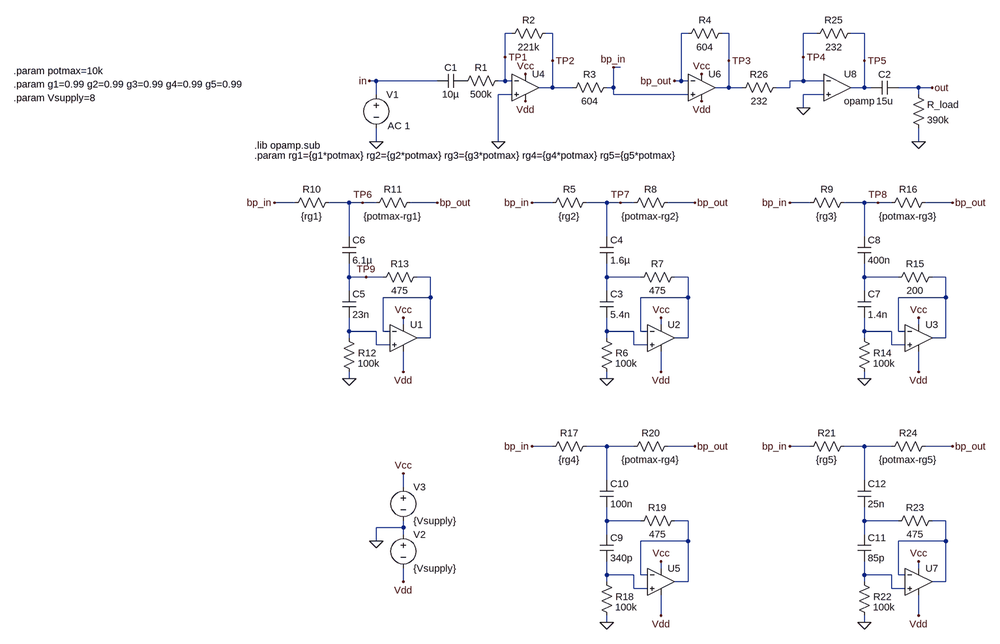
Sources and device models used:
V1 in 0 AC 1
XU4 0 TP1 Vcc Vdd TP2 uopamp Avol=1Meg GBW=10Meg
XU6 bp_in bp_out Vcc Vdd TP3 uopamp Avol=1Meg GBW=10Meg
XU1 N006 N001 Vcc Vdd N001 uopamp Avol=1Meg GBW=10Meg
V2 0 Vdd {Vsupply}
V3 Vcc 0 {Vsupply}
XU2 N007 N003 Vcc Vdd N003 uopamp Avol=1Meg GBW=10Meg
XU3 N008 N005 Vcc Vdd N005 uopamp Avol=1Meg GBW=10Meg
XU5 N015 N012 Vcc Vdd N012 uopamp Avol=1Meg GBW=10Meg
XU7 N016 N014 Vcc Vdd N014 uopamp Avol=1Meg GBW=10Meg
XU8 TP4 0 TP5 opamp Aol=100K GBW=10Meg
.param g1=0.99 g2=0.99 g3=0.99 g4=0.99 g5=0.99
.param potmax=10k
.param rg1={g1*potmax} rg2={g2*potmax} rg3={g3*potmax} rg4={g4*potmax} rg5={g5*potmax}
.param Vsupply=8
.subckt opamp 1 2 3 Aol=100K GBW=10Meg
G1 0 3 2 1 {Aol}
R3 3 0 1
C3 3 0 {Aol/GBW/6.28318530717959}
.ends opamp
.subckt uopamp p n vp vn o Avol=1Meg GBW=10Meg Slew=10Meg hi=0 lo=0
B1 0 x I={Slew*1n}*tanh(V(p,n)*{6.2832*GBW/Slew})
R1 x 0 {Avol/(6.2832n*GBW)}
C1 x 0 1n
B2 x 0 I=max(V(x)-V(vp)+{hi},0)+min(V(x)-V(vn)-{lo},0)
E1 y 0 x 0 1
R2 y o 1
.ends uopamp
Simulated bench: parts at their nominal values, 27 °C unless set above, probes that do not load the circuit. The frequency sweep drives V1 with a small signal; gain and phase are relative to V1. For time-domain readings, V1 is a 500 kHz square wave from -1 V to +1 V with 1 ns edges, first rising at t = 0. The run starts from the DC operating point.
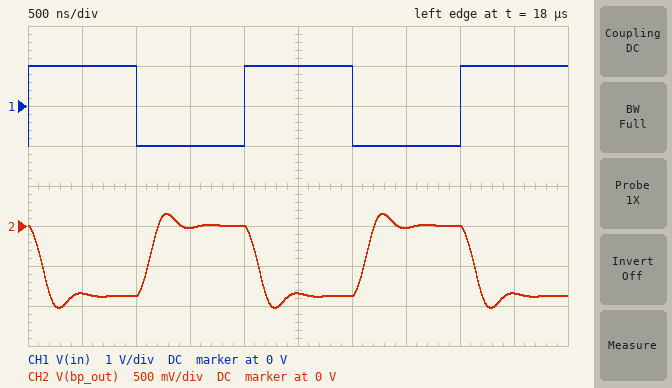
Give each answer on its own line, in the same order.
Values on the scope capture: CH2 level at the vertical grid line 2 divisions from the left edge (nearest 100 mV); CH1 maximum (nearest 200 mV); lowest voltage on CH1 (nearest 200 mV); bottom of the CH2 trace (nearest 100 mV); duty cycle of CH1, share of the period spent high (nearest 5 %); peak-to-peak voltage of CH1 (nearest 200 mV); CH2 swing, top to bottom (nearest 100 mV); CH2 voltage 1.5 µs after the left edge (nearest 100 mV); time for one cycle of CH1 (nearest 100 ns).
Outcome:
-900 mV
1.0 V
-1.0 V
-1.0 V
50 %
2.0 V
1.2 V
0 V
2.0 µs
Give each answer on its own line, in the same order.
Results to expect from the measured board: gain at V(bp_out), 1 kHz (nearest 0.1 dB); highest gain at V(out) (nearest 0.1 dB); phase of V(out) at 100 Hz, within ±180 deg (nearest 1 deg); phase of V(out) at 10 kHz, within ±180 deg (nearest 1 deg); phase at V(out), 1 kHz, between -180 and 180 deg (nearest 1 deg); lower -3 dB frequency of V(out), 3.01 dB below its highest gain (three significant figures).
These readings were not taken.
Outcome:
-7.2 dB
3.3 dB
5 deg
-10 deg
20 deg
836 Hz
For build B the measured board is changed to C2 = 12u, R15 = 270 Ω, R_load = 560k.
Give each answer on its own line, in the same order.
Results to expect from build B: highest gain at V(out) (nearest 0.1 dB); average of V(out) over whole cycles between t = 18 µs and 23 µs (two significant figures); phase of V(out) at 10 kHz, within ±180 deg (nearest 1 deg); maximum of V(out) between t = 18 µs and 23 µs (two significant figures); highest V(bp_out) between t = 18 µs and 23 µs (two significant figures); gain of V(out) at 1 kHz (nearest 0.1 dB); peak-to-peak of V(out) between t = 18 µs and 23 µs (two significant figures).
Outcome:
2.2 dB
1.0 V
-8 deg
2.0 V
140 mV
1.5 dB
1.9 V
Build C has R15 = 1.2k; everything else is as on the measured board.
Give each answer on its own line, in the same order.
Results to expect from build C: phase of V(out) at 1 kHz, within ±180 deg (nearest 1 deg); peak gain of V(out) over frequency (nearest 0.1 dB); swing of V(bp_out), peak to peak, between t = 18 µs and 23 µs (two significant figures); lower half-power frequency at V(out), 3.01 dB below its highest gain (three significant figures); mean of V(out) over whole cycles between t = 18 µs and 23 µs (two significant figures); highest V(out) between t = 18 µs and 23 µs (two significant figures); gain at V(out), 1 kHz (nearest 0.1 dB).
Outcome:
-6 deg
0.4 dB
1.1 V
30.6 Hz
940 mV
1.8 V
-2.7 dB
